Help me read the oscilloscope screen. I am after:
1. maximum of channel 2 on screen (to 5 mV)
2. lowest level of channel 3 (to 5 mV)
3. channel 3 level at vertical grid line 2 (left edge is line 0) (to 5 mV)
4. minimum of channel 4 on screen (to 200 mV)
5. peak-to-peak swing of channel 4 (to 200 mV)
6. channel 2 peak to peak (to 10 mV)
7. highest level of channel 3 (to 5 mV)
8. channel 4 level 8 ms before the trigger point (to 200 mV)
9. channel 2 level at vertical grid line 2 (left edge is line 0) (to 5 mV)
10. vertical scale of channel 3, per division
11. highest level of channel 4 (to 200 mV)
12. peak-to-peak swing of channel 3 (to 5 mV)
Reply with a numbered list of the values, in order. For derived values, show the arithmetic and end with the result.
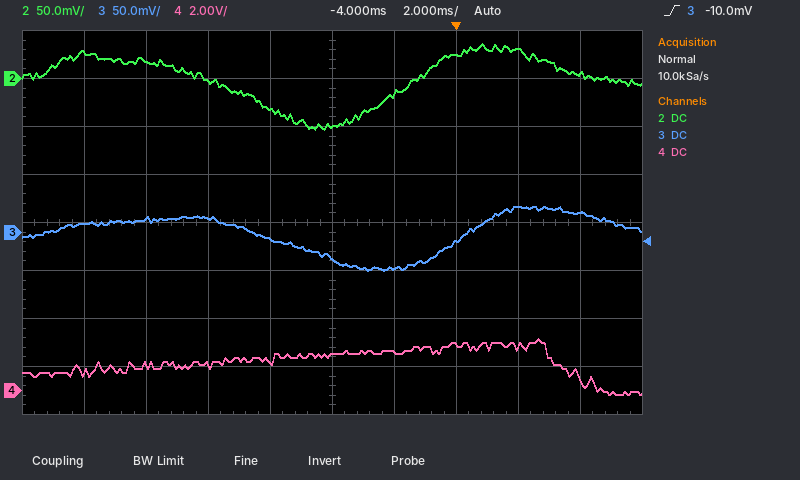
1. 35 mV
2. -40 mV
3. 15 mV
4. -200 mV
5. 2.2 V − (-200 mV) = 2.4 V
6. 90 mV
7. 25 mV
8. 1.0 V
9. 20 mV
10. 50 mV
11. 2.2 V
12. 25 mV − (-40 mV) = 65 mV
